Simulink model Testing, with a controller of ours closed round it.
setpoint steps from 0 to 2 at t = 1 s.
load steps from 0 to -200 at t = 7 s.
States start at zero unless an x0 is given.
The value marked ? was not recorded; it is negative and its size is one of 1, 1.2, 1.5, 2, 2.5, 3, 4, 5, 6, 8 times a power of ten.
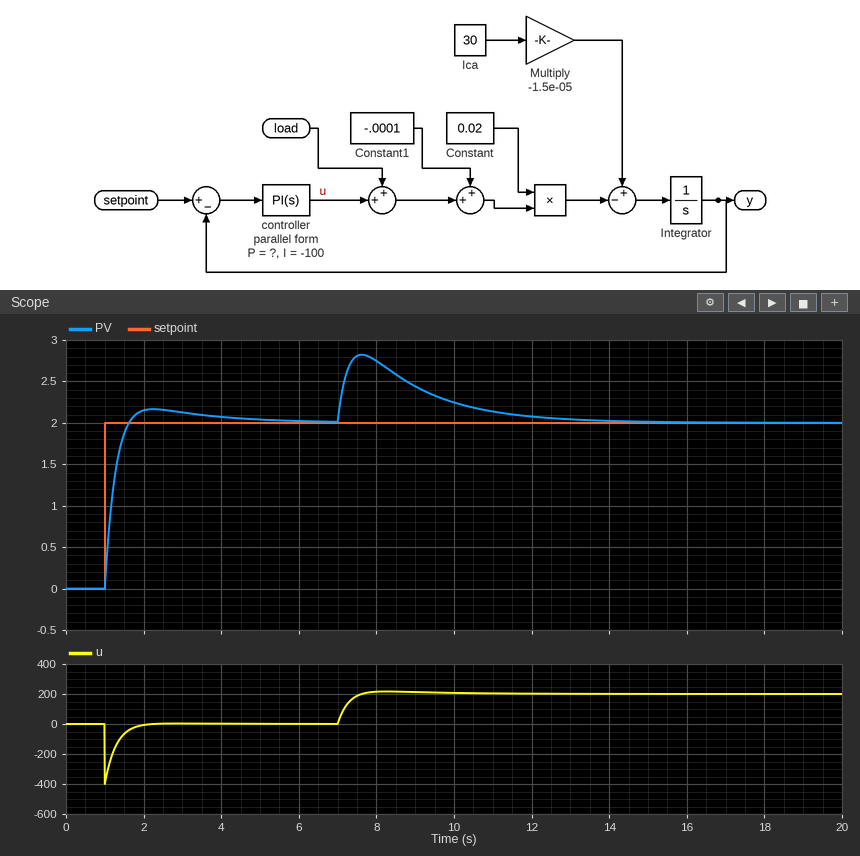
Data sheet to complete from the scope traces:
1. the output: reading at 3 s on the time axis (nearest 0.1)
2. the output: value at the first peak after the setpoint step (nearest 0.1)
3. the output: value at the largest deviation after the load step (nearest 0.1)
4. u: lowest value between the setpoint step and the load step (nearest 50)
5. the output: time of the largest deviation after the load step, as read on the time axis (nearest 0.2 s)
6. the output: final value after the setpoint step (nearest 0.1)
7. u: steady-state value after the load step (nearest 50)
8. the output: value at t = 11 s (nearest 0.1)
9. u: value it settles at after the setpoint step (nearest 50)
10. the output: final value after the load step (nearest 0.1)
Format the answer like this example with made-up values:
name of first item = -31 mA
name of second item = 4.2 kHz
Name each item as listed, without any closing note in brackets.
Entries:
the output: reading at 3 s on the time axis = 2.1
the output: value at the first peak after the setpoint step = 2.2
the output: value at the largest deviation after the load step = 2.8
u: lowest value between the setpoint step and the load step = -400
the output: time of the largest deviation after the load step, as read on the time axis = 7.6 s
the output: final value after the setpoint step = 2.0
u: steady-state value after the load step = 200
the output: value at t = 11 s = 2.1
u: value it settles at after the setpoint step = 0
the output: final value after the load step = 2.0
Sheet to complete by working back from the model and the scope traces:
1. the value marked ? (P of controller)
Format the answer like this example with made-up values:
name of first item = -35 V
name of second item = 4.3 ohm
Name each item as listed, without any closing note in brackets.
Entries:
the value marked ? = -200
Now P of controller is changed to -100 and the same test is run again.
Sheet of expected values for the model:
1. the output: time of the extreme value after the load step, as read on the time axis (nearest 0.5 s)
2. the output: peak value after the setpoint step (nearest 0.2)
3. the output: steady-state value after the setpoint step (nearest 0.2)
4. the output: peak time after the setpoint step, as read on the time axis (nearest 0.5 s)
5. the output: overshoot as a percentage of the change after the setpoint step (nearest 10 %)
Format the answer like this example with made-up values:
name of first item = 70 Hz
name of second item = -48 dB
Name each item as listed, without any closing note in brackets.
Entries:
the output: time of the extreme value after the load step, as read on the time axis = 8.0 s
the output: peak value after the setpoint step = 2.4
the output: steady-state value after the setpoint step = 2.0
the output: peak time after the setpoint step, as read on the time axis = 2.5 s
the output: overshoot as a percentage of the change after the setpoint step = 20 %
